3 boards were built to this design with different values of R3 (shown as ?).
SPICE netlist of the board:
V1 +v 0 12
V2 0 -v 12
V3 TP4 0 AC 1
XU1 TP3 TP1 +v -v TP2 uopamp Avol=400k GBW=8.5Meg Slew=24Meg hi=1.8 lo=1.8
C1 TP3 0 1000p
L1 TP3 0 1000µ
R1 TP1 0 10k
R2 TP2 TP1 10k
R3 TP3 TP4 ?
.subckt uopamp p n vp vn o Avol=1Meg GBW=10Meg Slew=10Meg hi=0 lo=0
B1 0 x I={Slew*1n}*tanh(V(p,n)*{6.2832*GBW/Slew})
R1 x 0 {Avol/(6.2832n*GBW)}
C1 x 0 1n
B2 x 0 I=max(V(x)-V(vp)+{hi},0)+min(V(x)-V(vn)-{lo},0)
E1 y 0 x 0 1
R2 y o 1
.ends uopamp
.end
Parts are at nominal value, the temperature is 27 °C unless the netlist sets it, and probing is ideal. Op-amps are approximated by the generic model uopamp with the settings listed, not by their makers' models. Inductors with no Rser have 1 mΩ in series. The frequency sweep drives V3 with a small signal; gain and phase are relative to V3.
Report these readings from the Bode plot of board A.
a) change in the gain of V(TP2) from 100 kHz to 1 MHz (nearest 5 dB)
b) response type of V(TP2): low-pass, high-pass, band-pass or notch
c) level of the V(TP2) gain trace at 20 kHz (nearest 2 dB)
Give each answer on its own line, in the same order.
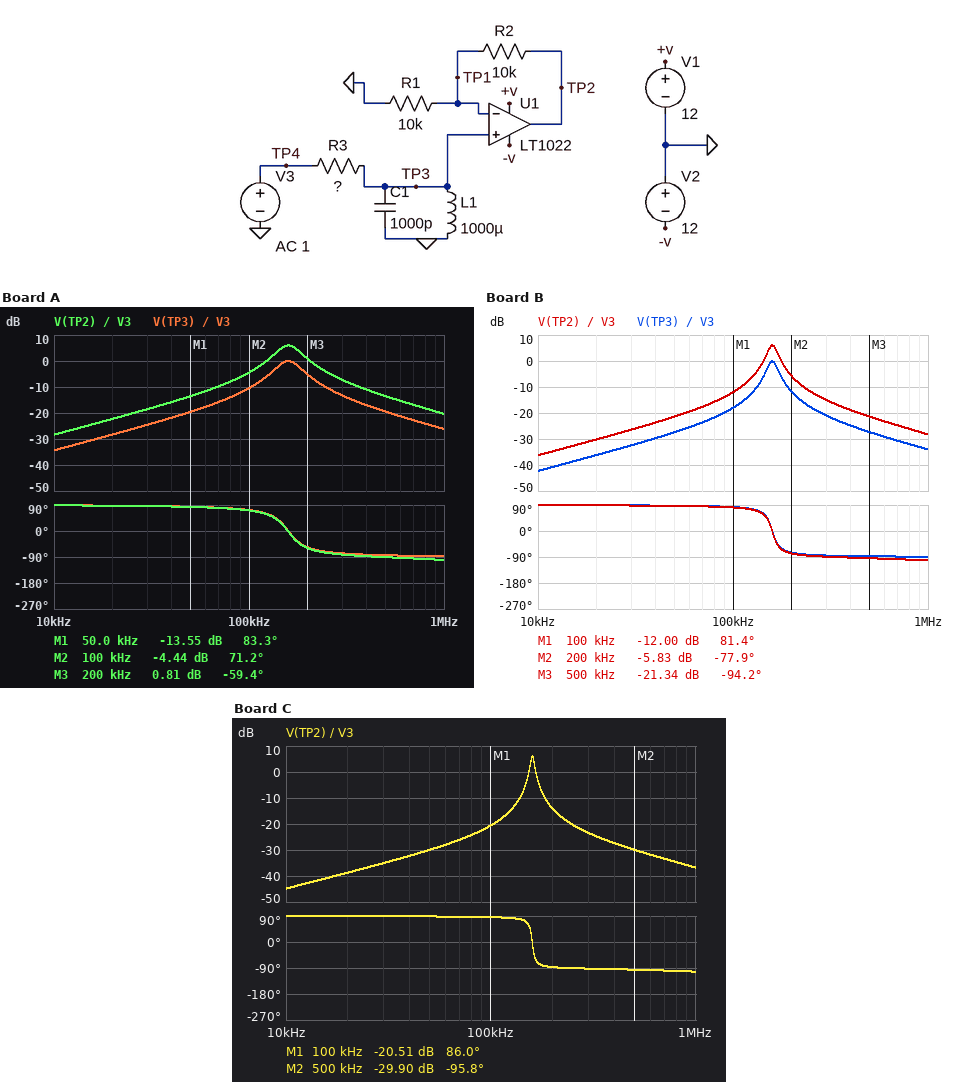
-15 dB
band-pass
-22 dB
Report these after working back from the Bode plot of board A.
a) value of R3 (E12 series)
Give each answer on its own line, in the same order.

3.3 kΩ
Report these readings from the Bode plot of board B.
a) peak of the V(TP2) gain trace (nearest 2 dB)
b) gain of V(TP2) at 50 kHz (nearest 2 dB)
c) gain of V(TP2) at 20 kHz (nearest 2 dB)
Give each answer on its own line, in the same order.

6 dB
-22 dB
-30 dB
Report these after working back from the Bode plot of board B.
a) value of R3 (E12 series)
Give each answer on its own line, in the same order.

8.2 kΩ
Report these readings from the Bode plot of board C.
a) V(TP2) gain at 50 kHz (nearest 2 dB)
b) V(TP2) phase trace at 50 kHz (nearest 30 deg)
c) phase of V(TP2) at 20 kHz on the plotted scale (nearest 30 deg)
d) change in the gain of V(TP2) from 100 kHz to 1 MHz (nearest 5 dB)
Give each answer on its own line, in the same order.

-30 dB
90 deg
90 deg
-15 dB
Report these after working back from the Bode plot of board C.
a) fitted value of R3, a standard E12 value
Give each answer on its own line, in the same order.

22 kΩ
